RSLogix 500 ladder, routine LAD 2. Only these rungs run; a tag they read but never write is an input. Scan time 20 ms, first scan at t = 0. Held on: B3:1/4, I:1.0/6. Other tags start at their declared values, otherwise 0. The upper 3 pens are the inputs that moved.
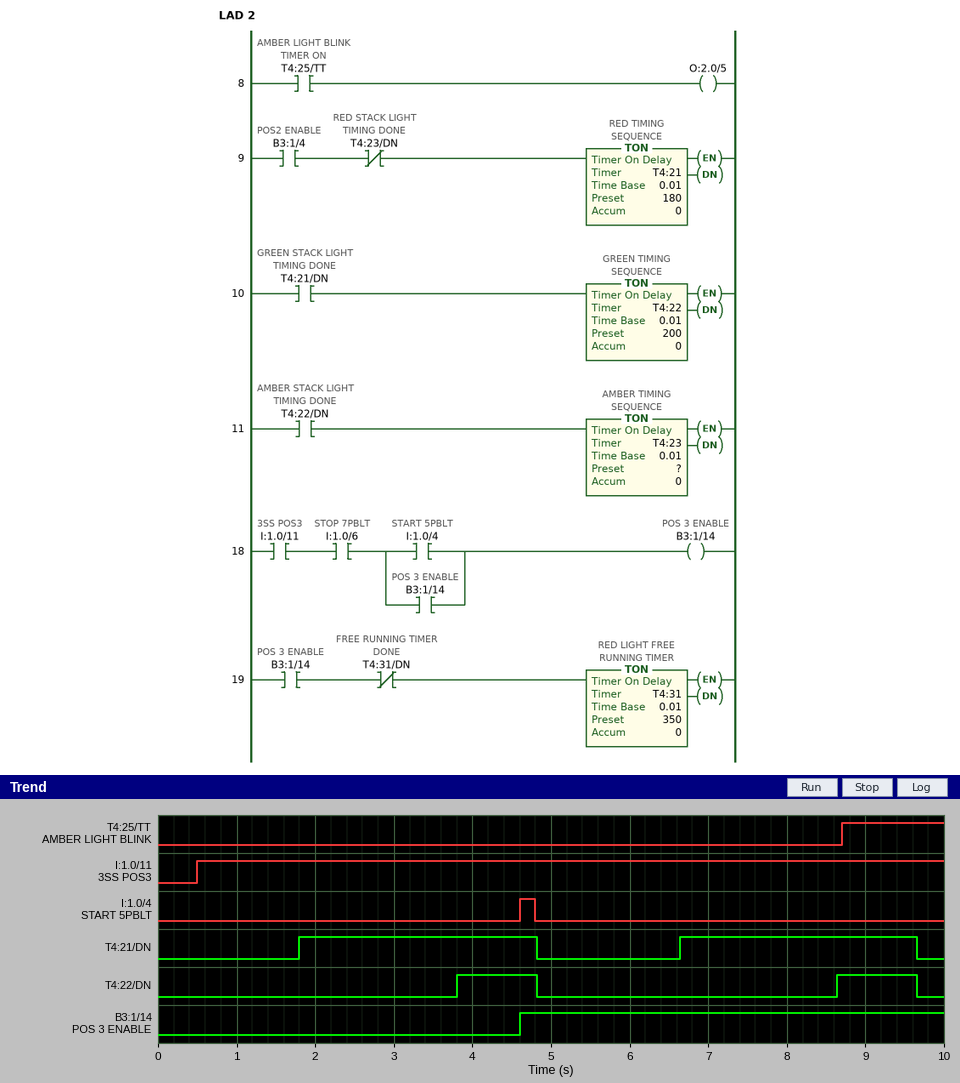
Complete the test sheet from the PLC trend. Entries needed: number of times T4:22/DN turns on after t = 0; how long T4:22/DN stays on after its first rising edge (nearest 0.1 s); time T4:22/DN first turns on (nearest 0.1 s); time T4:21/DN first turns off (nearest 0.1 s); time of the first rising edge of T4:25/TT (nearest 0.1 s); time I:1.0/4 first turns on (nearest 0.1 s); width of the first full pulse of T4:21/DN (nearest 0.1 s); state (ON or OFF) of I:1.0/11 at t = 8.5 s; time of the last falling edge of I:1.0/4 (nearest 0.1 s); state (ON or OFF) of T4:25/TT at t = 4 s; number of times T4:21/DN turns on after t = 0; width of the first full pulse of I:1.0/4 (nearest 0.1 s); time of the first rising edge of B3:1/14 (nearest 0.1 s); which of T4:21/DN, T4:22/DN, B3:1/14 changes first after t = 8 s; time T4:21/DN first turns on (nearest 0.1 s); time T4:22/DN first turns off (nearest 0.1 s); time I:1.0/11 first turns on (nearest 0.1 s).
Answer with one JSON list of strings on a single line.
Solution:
["2", "1.0 s", "3.8 s", "4.8 s", "8.7 s", "4.6 s", "3.0 s", "ON", "4.8 s", "OFF", "2", "0.2 s", "4.6 s", "T4:22/DN", "1.8 s", "4.8 s", "0.5 s"]
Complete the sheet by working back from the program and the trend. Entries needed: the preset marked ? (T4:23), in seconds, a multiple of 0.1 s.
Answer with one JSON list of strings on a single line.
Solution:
["1.0 s"]
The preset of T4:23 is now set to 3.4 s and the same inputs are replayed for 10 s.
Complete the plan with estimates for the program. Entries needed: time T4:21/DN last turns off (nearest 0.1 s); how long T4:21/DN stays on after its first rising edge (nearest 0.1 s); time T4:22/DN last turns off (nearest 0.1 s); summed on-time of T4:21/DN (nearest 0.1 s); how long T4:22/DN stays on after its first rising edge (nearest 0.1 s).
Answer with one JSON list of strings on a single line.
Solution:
["7.2 s", "5.4 s", "7.2 s", "6.4 s", "3.4 s"]
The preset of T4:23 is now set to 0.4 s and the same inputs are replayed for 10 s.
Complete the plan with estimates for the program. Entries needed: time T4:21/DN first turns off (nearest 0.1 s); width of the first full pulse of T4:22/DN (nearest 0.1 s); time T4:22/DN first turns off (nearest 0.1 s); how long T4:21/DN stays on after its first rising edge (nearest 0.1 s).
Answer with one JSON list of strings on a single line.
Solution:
["4.2 s", "0.4 s", "4.2 s", "2.4 s"]
